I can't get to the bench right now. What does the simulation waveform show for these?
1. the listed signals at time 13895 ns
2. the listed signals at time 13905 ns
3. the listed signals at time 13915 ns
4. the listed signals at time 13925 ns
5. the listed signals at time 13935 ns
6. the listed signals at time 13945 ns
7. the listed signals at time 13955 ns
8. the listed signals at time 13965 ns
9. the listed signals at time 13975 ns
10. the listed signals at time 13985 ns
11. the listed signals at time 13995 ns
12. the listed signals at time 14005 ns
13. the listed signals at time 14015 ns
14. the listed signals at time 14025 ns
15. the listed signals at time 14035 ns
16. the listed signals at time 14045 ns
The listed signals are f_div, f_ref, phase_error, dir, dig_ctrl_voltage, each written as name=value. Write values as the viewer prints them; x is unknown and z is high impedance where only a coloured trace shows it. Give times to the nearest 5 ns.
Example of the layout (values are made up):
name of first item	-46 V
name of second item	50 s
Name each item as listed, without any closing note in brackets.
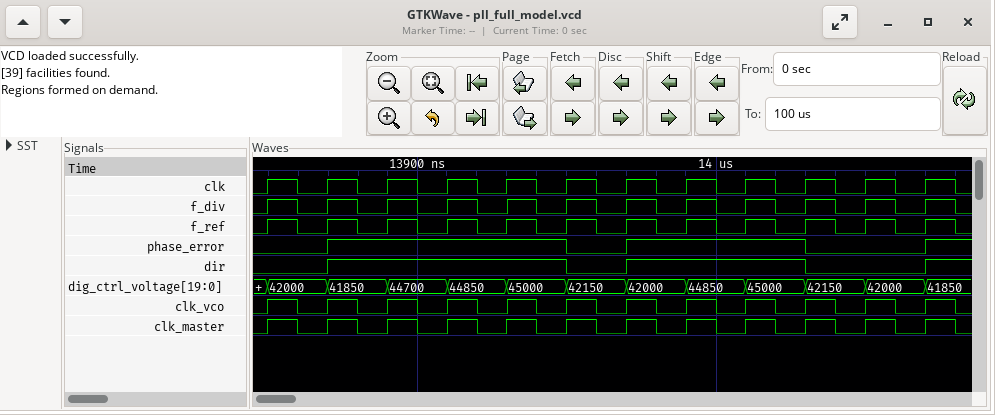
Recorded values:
the listed signals at time 13895 ns	f_div=1, f_ref=1, phase_error=1, dir=1, dig_ctrl_voltage=44700
the listed signals at time 13905 ns	f_div=0, f_ref=0, phase_error=1, dir=1, dig_ctrl_voltage=44700
the listed signals at time 13915 ns	f_div=1, f_ref=1, phase_error=1, dir=1, dig_ctrl_voltage=44850
the listed signals at time 13925 ns	f_div=0, f_ref=0, phase_error=1, dir=1, dig_ctrl_voltage=44850
the listed signals at time 13935 ns	f_div=1, f_ref=1, phase_error=1, dir=1, dig_ctrl_voltage=45000
the listed signals at time 13945 ns	f_div=0, f_ref=0, phase_error=1, dir=1, dig_ctrl_voltage=45000
the listed signals at time 13955 ns	f_div=1, f_ref=1, phase_error=0, dir=0, dig_ctrl_voltage=42150
the listed signals at time 13965 ns	f_div=0, f_ref=0, phase_error=0, dir=0, dig_ctrl_voltage=42150
the listed signals at time 13975 ns	f_div=1, f_ref=1, phase_error=1, dir=1, dig_ctrl_voltage=42000
the listed signals at time 13985 ns	f_div=0, f_ref=0, phase_error=1, dir=1, dig_ctrl_voltage=42000
the listed signals at time 13995 ns	f_div=1, f_ref=1, phase_error=1, dir=1, dig_ctrl_voltage=44850
the listed signals at time 14005 ns	f_div=0, f_ref=0, phase_error=1, dir=1, dig_ctrl_voltage=44850
the listed signals at time 14015 ns	f_div=1, f_ref=1, phase_error=1, dir=1, dig_ctrl_voltage=45000
the listed signals at time 14025 ns	f_div=0, f_ref=0, phase_error=1, dir=1, dig_ctrl_voltage=45000
the listed signals at time 14035 ns	f_div=1, f_ref=1, phase_error=0, dir=0, dig_ctrl_voltage=42150
the listed signals at time 14045 ns	f_div=0, f_ref=0, phase_error=0, dir=0, dig_ctrl_voltage=42150
